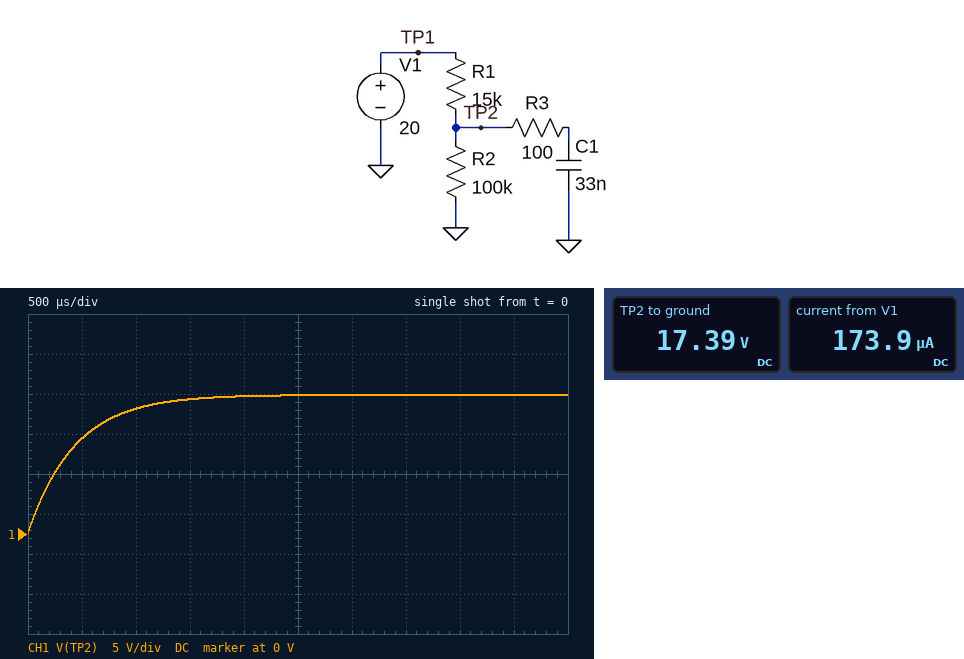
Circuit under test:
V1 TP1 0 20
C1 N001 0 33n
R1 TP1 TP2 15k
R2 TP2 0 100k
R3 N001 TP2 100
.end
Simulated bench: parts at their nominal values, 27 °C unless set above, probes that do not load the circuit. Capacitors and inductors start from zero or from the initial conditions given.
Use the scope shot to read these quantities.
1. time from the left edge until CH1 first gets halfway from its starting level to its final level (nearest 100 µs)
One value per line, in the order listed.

300 µs
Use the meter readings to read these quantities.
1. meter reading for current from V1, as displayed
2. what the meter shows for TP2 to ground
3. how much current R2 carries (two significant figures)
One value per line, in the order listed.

173.9 µA
17.39 V
170 µA
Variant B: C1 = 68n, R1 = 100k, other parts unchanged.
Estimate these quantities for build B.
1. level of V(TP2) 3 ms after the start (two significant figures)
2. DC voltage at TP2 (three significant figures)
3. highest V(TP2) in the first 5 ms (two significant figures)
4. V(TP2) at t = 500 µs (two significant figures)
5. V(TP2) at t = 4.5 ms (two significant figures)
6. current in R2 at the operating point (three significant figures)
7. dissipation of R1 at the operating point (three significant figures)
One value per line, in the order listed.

5.9 V
10.0 V
7.7 V
1.4 V
7.3 V
100 µA
1.00 mW
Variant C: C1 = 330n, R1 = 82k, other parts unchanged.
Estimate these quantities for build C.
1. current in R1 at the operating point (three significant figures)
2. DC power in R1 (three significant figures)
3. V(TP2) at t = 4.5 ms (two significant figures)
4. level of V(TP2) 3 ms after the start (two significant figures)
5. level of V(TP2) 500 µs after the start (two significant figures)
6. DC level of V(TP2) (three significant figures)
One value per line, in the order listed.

110 µA
990 µW
2.9 V
2.0 V
390 mV
11.0 V
